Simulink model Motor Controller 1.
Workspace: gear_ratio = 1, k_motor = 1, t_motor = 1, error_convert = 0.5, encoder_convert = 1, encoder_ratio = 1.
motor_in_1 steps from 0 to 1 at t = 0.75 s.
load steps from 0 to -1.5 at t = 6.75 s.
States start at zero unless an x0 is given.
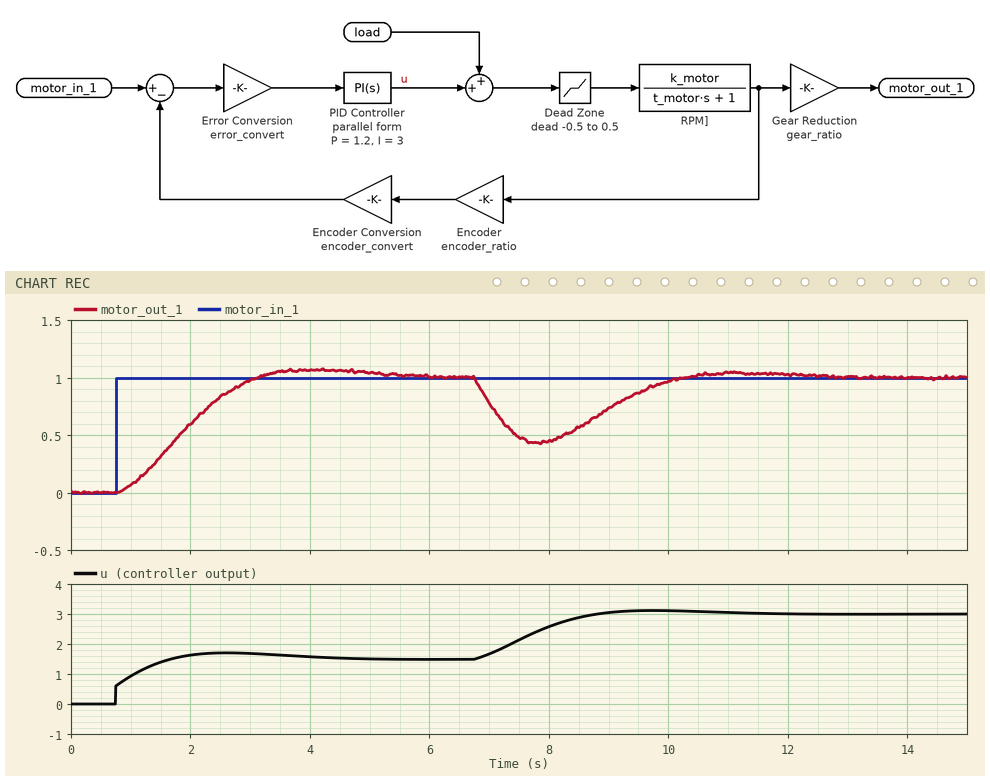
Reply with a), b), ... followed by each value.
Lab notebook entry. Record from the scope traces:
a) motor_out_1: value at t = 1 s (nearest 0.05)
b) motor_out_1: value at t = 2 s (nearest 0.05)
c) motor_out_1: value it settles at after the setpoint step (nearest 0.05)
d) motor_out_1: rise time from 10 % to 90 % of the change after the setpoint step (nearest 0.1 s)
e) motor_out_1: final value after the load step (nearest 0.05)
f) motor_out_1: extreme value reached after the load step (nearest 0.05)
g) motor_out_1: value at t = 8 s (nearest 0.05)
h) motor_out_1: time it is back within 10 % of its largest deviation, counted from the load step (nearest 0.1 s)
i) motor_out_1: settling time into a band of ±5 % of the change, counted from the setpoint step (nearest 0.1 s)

a) 0.05
b) 0.60
c) 1.00
d) 1.6 s
e) 1.00
f) 0.45
g) 0.45
h) 3.1 s
i) 4.0 s
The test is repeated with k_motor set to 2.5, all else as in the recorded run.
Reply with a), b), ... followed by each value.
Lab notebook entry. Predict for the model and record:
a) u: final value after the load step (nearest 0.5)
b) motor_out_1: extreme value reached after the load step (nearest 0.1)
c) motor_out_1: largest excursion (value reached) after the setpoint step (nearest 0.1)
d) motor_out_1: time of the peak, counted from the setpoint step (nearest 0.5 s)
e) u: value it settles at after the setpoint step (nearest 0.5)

a) 2.5
b) 0.3
c) 1.1
d) 2.0 s
e) 1.0
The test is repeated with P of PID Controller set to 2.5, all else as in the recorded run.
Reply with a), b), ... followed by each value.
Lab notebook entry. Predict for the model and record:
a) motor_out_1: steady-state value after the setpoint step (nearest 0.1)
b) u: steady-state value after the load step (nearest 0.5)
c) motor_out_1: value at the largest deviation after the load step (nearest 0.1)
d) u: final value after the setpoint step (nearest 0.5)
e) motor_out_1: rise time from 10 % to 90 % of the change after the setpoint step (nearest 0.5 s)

a) 1.0
b) 3.0
c) 0.5
d) 1.5
e) 2.0 s
